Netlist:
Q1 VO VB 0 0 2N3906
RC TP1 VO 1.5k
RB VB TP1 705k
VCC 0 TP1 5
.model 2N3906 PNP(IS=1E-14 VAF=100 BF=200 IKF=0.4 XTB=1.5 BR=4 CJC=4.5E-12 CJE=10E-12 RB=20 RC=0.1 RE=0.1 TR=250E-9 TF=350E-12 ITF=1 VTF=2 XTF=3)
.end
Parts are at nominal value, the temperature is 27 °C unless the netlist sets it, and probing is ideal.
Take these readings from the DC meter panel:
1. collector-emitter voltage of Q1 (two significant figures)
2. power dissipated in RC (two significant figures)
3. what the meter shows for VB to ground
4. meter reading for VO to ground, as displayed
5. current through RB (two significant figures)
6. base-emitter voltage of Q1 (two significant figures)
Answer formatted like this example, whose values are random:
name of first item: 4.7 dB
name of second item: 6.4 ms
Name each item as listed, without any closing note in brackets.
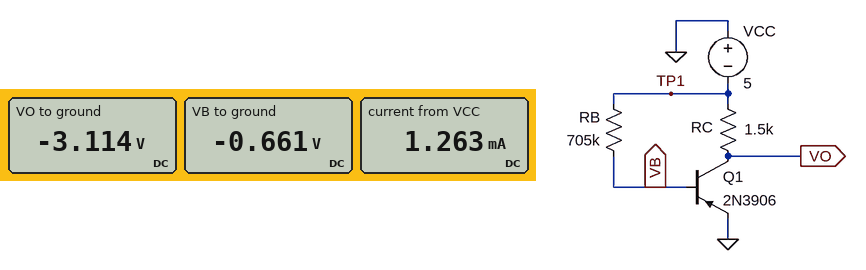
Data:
collector-emitter voltage of Q1: -3.1 V
power dissipated in RC: 2.4 mW
what the meter shows for VB to ground: -0.661 V
meter reading for VO to ground, as displayed: -3.114 V
current through RB: 6.2 µA
base-emitter voltage of Q1: -660 mV
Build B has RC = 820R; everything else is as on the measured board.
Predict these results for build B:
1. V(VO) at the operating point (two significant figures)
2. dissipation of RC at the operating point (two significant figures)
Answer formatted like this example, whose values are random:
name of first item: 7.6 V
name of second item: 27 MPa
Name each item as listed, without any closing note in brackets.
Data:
V(VO) at the operating point: -4.0 V
dissipation of RC at the operating point: 1.3 mW
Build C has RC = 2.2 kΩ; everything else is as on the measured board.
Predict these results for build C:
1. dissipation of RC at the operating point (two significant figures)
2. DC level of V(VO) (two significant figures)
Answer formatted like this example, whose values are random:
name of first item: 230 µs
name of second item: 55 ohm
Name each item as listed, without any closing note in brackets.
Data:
dissipation of RC at the operating point: 3.4 mW
DC level of V(VO): -2.3 V
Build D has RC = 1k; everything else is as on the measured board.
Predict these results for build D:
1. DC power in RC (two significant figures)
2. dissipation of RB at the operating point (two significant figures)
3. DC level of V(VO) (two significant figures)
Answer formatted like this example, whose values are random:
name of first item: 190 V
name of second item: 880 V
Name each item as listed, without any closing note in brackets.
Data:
DC power in RC: 1.6 mW
dissipation of RB at the operating point: 27 µW
DC level of V(VO): -3.7 V
